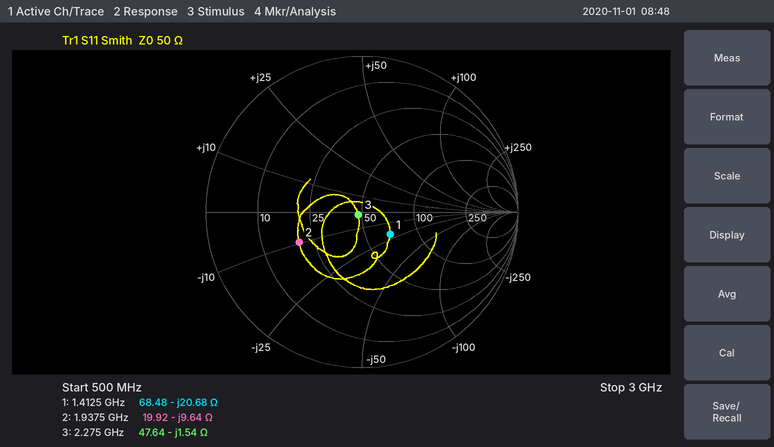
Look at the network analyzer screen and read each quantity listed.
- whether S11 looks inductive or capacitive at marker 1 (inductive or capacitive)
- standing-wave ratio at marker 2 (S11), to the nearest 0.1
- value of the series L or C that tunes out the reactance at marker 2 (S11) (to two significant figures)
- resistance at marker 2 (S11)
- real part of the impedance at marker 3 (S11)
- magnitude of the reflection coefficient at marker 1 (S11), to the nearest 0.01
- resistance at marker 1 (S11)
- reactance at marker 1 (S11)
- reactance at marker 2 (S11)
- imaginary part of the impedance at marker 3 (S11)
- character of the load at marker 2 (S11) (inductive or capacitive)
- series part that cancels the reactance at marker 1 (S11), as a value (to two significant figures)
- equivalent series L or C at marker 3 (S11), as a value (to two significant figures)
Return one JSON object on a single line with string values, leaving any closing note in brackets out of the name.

{"whether S11 looks inductive or capacitive at marker 1": "capacitive", "standing-wave ratio at marker 2 (S11), to the nearest 0.1": "2.6", "value of the series L or C that tunes out the reactance at marker 2 (S11)": "790 pH", "resistance at marker 2": "19.92 Ω", "real part of the impedance at marker 3": "47.64 Ω", "magnitude of the reflection coefficient at marker 1 (S11), to the nearest 0.01": "0.23", "resistance at marker 1": "68.48 Ω", "reactance at marker 1": "-20.68 Ω", "reactance at marker 2": "-9.64 Ω", "imaginary part of the impedance at marker 3": "-1.54 Ω", "character of the load at marker 2 (S11)": "capacitive", "series part that cancels the reactance at marker 1 (S11), as a value": "2.3 nH", "equivalent series L or C at marker 3 (S11), as a value": "45 pF"}
